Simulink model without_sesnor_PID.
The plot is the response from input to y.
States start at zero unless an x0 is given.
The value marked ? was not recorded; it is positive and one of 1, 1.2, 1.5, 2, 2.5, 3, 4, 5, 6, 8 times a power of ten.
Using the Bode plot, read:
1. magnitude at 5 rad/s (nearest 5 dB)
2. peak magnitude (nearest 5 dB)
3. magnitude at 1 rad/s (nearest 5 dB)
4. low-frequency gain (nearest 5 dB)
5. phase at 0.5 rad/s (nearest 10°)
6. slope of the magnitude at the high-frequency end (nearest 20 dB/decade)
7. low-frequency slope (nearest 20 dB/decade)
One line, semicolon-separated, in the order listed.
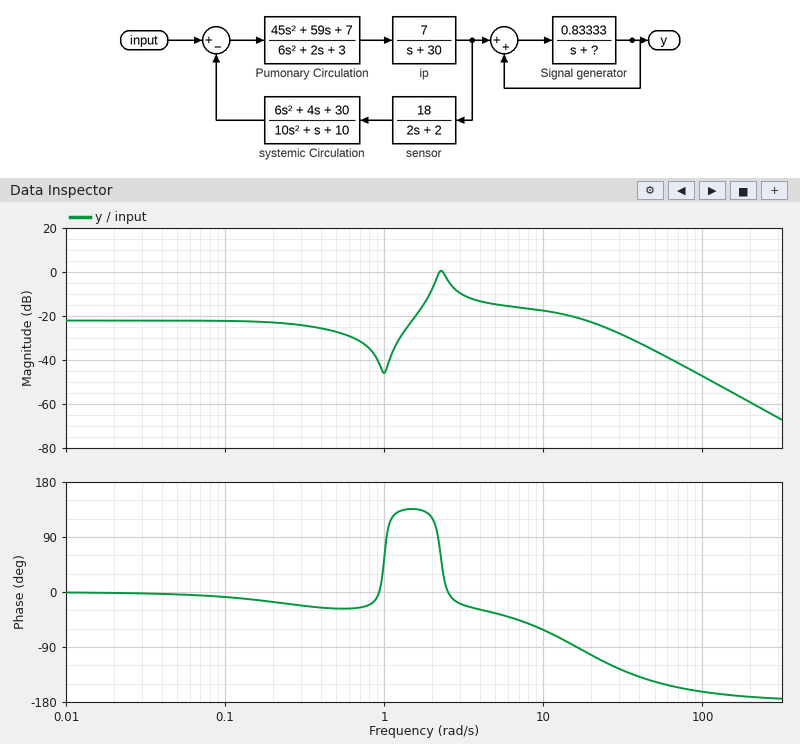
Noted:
-15 dB; 0 dB; -45 dB; -20 dB; -30°; -40 dB/decade; 0 dB/decade
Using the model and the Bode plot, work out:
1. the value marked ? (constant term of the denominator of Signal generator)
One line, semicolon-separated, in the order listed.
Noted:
1.2
